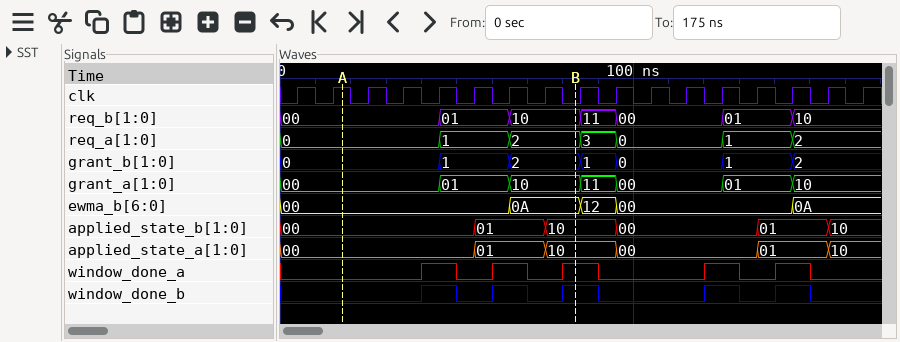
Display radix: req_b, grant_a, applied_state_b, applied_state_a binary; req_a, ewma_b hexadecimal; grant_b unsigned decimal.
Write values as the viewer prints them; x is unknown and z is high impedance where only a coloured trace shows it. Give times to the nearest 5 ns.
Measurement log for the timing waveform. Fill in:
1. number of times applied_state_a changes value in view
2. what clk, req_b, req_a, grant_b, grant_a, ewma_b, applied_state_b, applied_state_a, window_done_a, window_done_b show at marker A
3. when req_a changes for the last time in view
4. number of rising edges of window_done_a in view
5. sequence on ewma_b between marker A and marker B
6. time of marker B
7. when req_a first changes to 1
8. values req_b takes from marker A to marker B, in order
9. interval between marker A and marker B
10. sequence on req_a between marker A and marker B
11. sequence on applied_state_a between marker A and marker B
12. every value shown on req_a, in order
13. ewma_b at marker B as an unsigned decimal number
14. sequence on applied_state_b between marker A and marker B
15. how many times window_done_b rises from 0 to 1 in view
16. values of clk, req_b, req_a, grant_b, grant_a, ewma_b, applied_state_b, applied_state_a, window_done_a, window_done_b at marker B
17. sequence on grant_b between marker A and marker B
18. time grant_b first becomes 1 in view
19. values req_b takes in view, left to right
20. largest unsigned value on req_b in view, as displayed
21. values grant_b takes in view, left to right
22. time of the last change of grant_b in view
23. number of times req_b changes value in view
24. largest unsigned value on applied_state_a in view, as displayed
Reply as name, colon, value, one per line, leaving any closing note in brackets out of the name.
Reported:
number of times applied_state_a changes value in view: 5
what clk, req_b, req_a, grant_b, grant_a, ewma_b, applied_state_b, applied_state_a, window_done_a, window_done_b show at marker A: clk=1, req_b=00, req_a=0, grant_b=0, grant_a=00, ewma_b=00, applied_state_b=00, applied_state_a=00, window_done_a=0, window_done_b=0
when req_a changes for the last time in view: 145 ns
number of rising edges of window_done_a in view: 5
sequence on ewma_b between marker A and marker B: 00, 0A
time of marker B: 85 ns
when req_a first changes to 1: 45 ns
values req_b takes from marker A to marker B, in order: 00, 01, 10
interval between marker A and marker B: 65 ns
sequence on req_a between marker A and marker B: 0, 1, 2
sequence on applied_state_a between marker A and marker B: 00, 01, 10
every value shown on req_a, in order: 0, 1, 2, 3, 0, 1, 2
ewma_b at marker B as an unsigned decimal number: 10
sequence on applied_state_b between marker A and marker B: 00, 01, 10
how many times window_done_b rises from 0 to 1 in view: 5
values of clk, req_b, req_a, grant_b, grant_a, ewma_b, applied_state_b, applied_state_a, window_done_a, window_done_b at marker B: clk=0, req_b=10, req_a=2, grant_b=2, grant_a=10, ewma_b=0A, applied_state_b=10, applied_state_a=10, window_done_a=1, window_done_b=1
sequence on grant_b between marker A and marker B: 0, 1, 2
time grant_b first becomes 1 in view: 45 ns
values req_b takes in view, left to right: 00, 01, 10, 11, 00, 01, 10
largest unsigned value on req_b in view, as displayed: 11
values grant_b takes in view, left to right: 0, 1, 2, 1, 0, 1, 2
time of the last change of grant_b in view: 145 ns
number of times req_b changes value in view: 6
largest unsigned value on applied_state_a in view, as displayed: 10
